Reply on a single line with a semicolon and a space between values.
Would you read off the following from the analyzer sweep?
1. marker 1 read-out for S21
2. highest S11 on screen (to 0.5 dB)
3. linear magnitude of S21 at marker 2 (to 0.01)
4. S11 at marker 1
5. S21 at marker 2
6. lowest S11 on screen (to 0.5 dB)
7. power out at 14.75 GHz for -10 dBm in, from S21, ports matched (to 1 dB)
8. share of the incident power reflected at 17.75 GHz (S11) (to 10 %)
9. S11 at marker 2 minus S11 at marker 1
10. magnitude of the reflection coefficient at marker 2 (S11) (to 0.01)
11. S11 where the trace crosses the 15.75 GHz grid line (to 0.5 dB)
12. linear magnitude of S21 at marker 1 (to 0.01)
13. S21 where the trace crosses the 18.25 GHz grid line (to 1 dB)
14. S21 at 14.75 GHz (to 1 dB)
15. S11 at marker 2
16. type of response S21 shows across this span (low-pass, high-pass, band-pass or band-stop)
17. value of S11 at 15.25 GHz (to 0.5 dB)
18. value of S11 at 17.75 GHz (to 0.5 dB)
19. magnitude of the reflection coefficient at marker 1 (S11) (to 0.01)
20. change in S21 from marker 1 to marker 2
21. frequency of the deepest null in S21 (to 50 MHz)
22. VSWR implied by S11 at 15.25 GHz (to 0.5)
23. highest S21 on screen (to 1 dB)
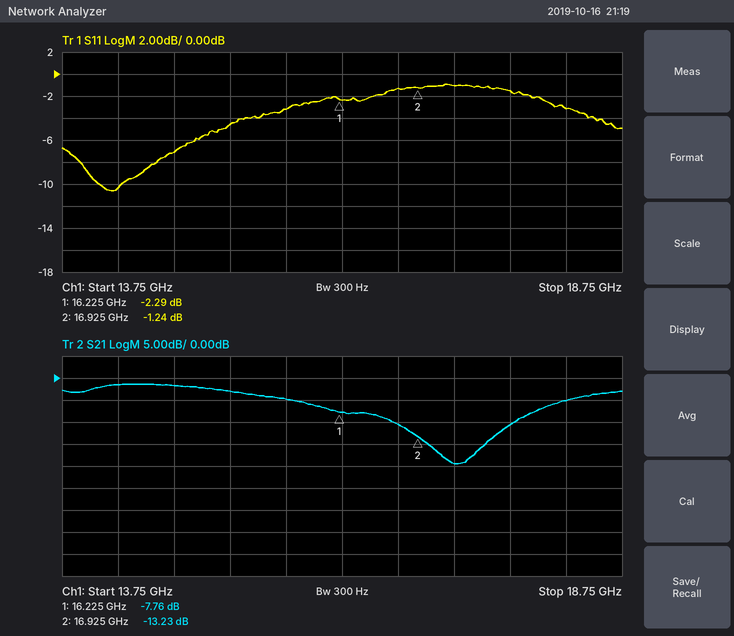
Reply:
-7.76 dB; -1.0 dB; 0.22; -2.29 dB; -13.23 dB; -10.5 dB; -12 dBm; 70 %; 1.05 dB; 0.87; -3.0 dB; 0.41; -5 dB; -2 dB; -1.24 dB; band-stop; -4.5 dB; -1.5 dB; 0.77; -5.47 dB; 17.25 GHz; 4.0; -1 dB
